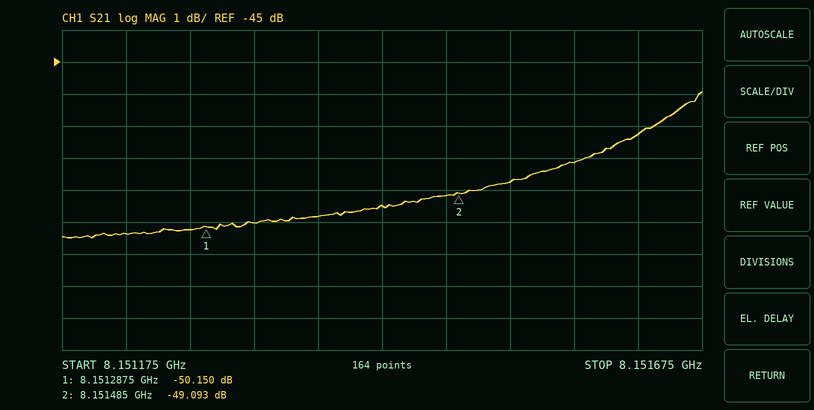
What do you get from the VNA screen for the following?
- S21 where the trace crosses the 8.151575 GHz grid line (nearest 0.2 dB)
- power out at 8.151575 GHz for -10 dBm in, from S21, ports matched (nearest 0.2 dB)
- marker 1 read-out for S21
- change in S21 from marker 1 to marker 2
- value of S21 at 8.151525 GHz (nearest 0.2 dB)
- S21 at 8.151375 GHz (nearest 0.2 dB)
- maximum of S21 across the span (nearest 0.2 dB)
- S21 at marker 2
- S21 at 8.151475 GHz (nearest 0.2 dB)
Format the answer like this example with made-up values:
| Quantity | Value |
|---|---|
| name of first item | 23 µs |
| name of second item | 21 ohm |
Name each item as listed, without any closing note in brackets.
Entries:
| Quantity | Value |
|---|---|
| S21 where the trace crosses the 8.151575 GHz grid line | -48.2 dB |
| power out at 8.151575 GHz for -10 dBm in, from S21, ports matched | -58.2 dBm |
| marker 1 read-out for S21 | -50.150 dB |
| change in S21 from marker 1 to marker 2 | 1.057 dB |
| value of S21 at 8.151525 GHz | -48.8 dB |
| S21 at 8.151375 GHz | -49.8 dB |
| maximum of S21 across the span | -46.0 dB |
| S21 at marker 2 | -49.093 dB |
| S21 at 8.151475 GHz | -49.2 dB |
